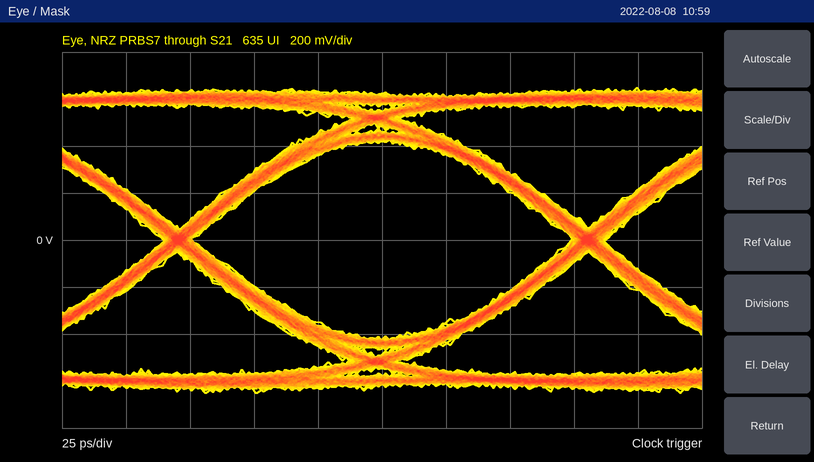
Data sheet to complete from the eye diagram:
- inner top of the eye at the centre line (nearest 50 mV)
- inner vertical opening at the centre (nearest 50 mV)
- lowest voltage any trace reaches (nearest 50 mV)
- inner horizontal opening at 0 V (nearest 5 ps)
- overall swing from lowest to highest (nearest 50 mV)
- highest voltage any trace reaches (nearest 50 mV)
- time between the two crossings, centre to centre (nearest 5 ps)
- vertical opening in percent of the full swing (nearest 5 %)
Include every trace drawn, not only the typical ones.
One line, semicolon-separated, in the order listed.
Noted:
400 mV; 850 mV; -650 mV; 150 ps; 1.30 V; 650 mV; 160 ps; 65 %
